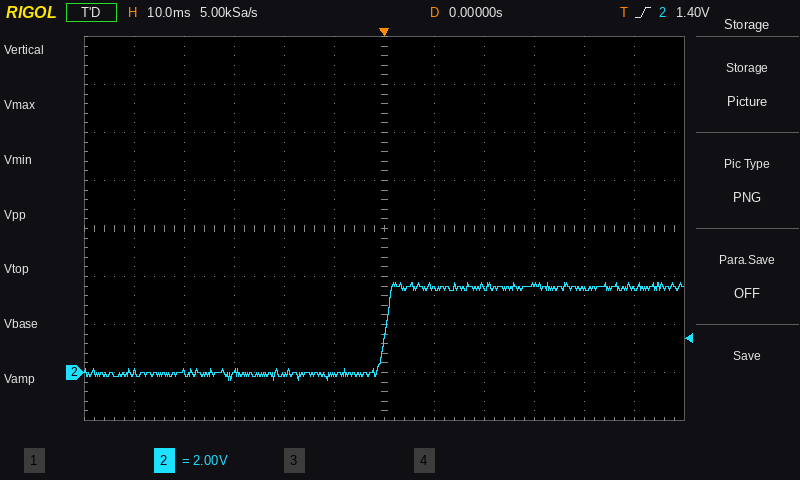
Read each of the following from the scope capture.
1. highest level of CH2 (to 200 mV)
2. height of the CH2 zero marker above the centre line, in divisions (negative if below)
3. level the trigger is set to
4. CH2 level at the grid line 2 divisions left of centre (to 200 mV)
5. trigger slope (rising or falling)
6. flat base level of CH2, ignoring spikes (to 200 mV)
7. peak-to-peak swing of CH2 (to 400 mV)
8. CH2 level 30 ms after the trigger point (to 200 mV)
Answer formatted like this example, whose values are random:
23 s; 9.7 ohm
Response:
3.8 V; -3.0 div; 1.40 V; 0.0 V; rising; 0.0 V; 4.0 V; 3.6 V
